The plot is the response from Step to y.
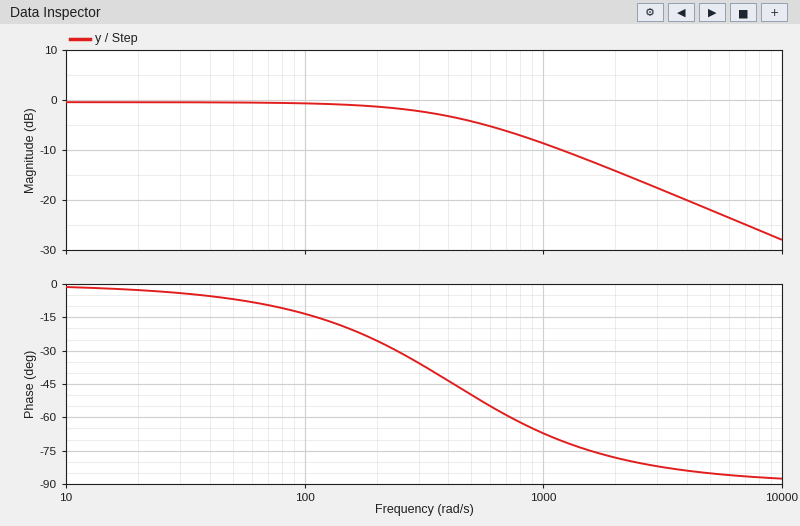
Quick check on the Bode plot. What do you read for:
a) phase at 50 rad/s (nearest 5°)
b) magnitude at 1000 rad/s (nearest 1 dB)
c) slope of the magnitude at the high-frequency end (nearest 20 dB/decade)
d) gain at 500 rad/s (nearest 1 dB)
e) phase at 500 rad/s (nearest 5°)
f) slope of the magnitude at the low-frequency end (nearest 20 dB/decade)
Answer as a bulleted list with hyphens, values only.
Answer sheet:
- -5°
- -9 dB
- -20 dB/decade
- -4 dB
- -50°
- 0 dB/decade
